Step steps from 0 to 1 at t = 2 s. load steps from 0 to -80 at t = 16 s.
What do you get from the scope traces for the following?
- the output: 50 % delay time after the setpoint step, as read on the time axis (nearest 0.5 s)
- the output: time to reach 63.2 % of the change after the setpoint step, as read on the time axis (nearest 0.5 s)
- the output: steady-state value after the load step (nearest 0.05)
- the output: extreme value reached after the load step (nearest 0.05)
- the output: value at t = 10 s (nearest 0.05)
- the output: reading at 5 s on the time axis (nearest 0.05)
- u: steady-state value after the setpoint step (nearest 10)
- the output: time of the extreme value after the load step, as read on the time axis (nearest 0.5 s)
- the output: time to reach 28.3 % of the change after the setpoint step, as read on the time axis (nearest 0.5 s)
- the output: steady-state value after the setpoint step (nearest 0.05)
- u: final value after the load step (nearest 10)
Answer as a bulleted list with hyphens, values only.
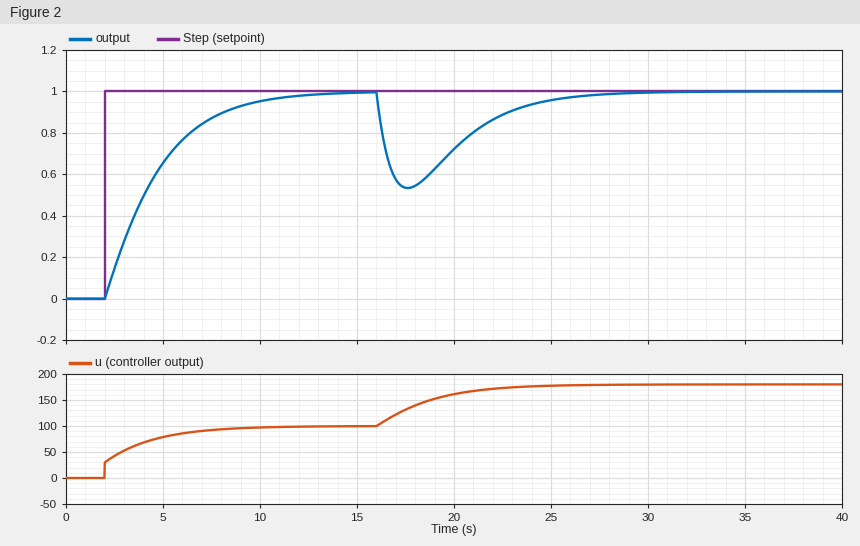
- 4.0 s
- 5.0 s
- 1.00
- 0.55
- 0.95
- 0.65
- 100
- 17.5 s
- 3.0 s
- 1.00
- 180
